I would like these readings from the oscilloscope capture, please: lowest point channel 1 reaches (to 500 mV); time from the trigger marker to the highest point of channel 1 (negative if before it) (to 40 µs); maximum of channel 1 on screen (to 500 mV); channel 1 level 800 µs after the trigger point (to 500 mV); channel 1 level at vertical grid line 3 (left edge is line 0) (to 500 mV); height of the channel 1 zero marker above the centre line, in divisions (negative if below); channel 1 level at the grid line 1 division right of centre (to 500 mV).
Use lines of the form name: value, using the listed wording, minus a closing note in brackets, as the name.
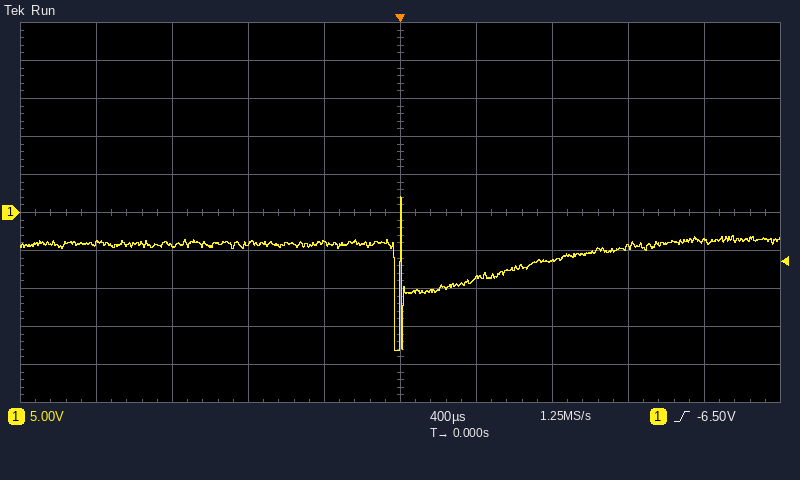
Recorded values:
lowest point channel 1 reaches: -18.0 V
time from the trigger marker to the highest point of channel 1 (negative if before it): 0 µs
maximum of channel 1 on screen: 2.0 V
channel 1 level 800 µs after the trigger point: -6.5 V
channel 1 level at vertical grid line 3 (left edge is line 0): -4.0 V
height of the channel 1 zero marker above the centre line, in divisions: 0.0 div
channel 1 level at the grid line 1 division right of centre: -8.5 V
